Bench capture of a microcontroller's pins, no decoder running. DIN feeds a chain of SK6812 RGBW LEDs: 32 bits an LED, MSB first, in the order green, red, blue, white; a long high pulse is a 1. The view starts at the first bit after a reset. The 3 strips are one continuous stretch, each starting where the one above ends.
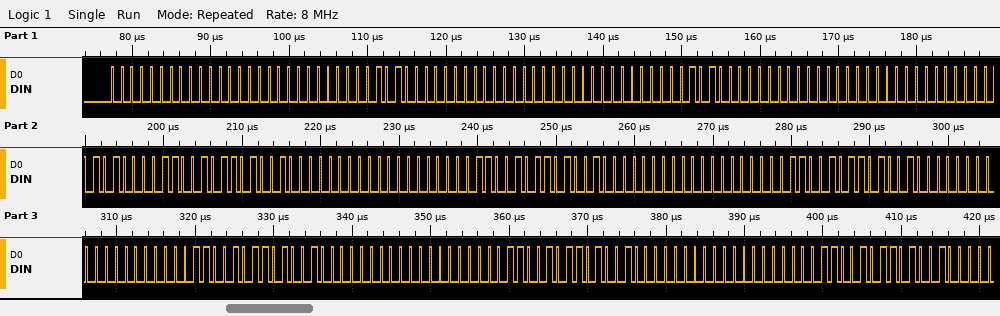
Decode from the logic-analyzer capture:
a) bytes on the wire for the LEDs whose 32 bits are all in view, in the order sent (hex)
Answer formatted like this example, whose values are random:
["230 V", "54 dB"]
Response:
["00 00 00 14 00 00 00 14 00 00 00 14 32 D2 00 00 32 D2 00 00 32 D2 00 00 32 D2 00 00 32 D2 00 00"]
